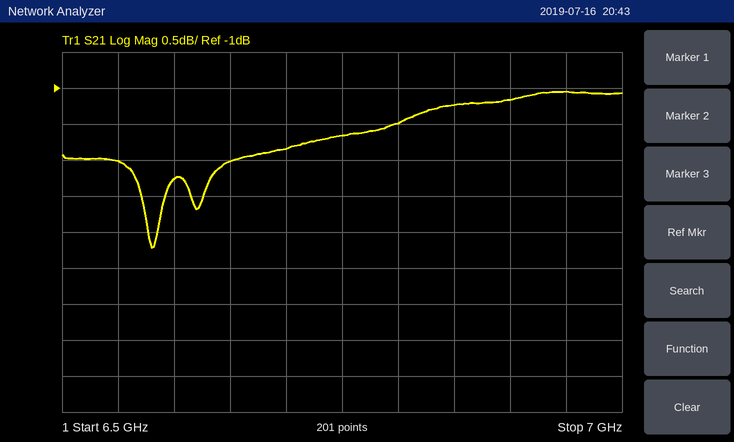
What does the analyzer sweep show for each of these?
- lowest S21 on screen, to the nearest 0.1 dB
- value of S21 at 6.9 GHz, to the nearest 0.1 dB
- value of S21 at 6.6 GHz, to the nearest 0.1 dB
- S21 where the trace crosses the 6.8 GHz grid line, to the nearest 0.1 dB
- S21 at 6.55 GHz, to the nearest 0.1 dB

-3.2 dB
-1.2 dB
-2.3 dB
-1.5 dB
-2.0 dB
